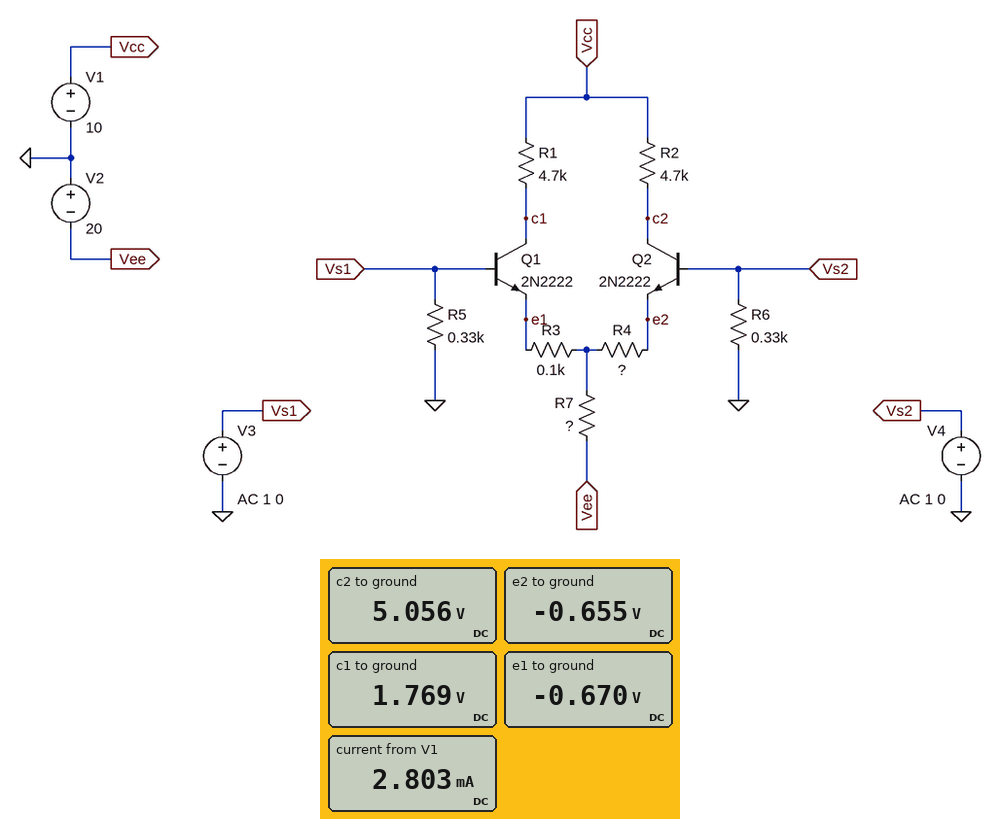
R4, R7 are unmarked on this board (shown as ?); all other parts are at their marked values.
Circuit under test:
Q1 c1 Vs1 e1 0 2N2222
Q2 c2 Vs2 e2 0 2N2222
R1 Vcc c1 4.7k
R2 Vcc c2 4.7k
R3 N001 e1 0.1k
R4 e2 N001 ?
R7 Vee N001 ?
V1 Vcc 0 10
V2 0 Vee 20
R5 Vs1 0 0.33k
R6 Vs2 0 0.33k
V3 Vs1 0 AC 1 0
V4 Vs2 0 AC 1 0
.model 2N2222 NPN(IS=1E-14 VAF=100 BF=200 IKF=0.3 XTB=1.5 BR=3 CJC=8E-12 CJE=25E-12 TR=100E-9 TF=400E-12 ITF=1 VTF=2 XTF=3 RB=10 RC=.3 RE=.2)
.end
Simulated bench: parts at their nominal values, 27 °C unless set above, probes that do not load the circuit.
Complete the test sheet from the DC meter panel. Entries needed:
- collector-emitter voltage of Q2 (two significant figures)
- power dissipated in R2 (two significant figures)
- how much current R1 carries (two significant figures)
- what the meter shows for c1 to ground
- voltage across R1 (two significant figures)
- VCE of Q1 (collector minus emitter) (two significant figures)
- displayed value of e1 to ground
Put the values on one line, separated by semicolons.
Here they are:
5.7 V; 5.2 mW; 1.8 mA; 1.769 V; 8.2 V; 2.4 V; -0.670 V
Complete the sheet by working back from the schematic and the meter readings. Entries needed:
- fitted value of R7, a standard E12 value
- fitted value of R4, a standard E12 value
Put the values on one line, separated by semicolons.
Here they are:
6.8 kΩ; 180 Ω
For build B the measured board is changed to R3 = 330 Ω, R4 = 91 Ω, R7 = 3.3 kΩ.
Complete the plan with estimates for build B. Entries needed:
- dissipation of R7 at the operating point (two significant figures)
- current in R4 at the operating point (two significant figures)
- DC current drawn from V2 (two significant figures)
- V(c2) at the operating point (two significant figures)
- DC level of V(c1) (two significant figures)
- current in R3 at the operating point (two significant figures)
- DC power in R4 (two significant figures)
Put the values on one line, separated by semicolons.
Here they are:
110 mW; 4.3 mA; 5.7 mA; -720 mV; 3.4 V; 1.4 mA; 1.7 mW
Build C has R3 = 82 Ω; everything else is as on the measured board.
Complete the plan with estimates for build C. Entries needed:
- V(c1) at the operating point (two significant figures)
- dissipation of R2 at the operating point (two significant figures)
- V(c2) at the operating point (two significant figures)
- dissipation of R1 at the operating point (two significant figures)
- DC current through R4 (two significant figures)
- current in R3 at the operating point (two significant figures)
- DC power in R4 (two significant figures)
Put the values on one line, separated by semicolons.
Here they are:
1.3 V; 4.2 mW; 5.5 V; 16 mW; 950 µA; 1.9 mA; 160 µW
